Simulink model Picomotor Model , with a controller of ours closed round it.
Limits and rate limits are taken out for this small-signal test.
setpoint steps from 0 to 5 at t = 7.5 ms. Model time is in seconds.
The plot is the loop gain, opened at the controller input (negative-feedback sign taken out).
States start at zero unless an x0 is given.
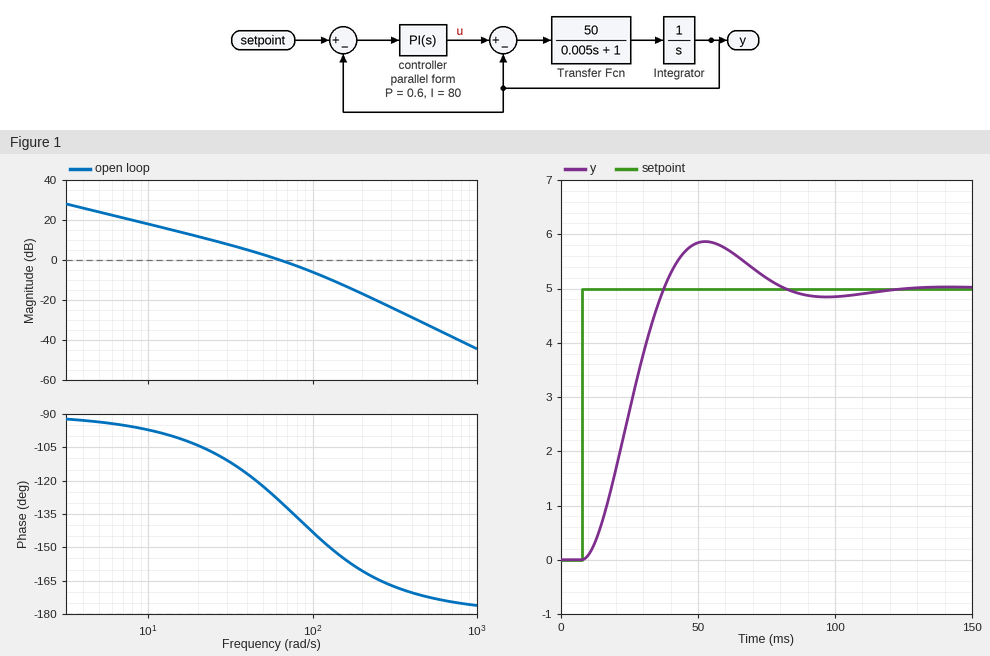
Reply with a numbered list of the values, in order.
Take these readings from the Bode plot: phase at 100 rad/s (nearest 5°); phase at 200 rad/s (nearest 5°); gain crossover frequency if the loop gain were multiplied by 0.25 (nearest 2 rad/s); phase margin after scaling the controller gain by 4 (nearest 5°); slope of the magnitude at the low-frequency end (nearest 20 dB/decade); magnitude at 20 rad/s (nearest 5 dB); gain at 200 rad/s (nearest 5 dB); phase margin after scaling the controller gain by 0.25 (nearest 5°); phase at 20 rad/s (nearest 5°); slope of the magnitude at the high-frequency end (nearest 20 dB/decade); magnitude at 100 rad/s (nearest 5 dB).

1. -145°
2. -160°
3. 20 rad/s
4. 25°
5. -20 dB/decade
6. 10 dB
7. -15 dB
8. 75°
9. -105°
10. -40 dB/decade
11. -5 dB
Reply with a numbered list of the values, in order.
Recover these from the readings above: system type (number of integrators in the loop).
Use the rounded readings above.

1. 1
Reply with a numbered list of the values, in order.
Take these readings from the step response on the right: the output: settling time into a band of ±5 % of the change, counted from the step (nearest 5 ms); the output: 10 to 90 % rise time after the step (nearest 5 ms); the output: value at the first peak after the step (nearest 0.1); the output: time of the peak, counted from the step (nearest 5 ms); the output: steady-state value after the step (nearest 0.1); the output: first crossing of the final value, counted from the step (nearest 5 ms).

1. 65 ms
2. 20 ms
3. 5.9
4. 45 ms
5. 5.0
6. 30 ms
